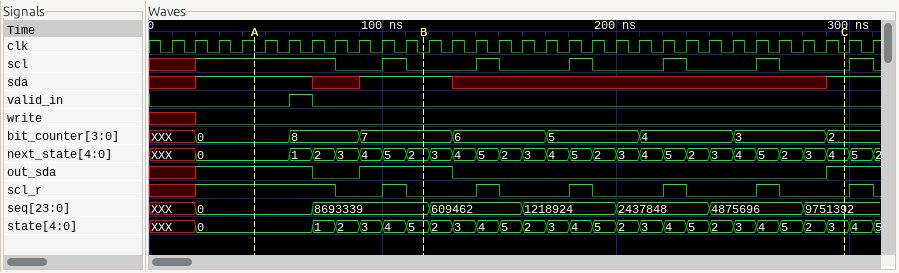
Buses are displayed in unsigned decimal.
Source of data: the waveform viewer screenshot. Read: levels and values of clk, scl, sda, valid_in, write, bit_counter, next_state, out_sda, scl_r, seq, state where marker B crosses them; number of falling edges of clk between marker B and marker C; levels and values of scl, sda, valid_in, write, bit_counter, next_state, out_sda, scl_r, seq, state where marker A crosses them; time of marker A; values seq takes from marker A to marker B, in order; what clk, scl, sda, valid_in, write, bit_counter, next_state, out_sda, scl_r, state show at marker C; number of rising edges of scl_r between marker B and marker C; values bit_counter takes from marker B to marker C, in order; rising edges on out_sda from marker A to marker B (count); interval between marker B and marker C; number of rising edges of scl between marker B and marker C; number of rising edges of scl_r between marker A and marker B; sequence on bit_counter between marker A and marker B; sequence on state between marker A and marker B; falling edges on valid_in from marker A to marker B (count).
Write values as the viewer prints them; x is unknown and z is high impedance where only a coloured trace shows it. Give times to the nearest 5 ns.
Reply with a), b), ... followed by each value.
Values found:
a) clk=0, scl=0, sda=1, valid_in=0, write=0, bit_counter=7, next_state=2, out_sda=1, scl_r=0, seq=8693339, state=5
b) 18
c) scl=1, sda=1, valid_in=0, write=0, bit_counter=0, next_state=0, out_sda=1, scl_r=1, seq=0, state=0
d) 45 ns
e) 0, 8693339
f) clk=0, scl=0, sda=1, valid_in=0, write=0, bit_counter=2, next_state=4, out_sda=1, scl_r=0, state=3
g) 4
h) 7, 6, 5, 4, 3, 2
i) 1
j) 180 ns
k) 4
l) 1
m) 0, 8, 7
n) 0, 1, 2, 3, 4, 5
o) 1
